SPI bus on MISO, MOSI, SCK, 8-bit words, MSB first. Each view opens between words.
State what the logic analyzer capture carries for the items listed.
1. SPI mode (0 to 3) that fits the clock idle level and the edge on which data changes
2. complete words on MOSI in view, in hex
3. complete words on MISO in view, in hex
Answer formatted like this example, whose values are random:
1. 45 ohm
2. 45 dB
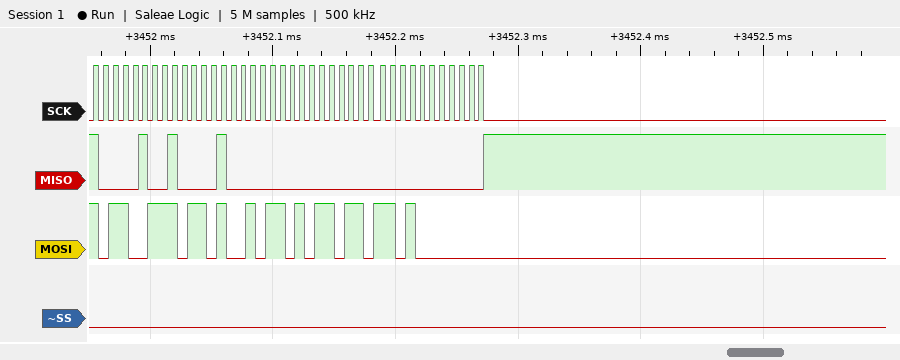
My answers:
1. 0
2. B3, B4, B5, B6, 80
3. 84, 84, 00, 00, 00
